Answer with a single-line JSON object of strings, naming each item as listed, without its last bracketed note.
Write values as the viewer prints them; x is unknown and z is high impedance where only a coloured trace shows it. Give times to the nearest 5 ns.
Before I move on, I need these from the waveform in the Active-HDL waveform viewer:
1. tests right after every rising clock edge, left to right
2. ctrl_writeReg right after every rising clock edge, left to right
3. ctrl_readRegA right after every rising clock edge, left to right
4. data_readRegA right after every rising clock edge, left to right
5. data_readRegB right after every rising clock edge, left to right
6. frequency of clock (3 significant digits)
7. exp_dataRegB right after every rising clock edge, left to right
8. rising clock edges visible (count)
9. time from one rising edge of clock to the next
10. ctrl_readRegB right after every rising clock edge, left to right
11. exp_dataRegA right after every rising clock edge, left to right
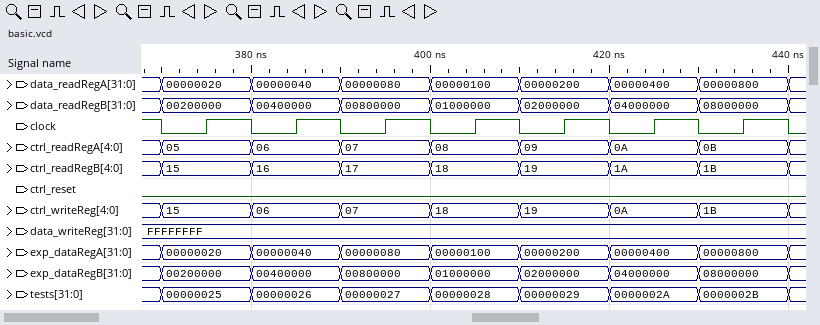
{"tests right after every rising clock edge, left to right": "00000025, 00000026, 00000027, 00000028, 00000029, 0000002A, 0000002B", "ctrl_writeReg right after every rising clock edge, left to right": "15, 06, 07, 18, 19, 0A, 1B", "ctrl_readRegA right after every rising clock edge, left to right": "05, 06, 07, 08, 09, 0A, 0B", "data_readRegA right after every rising clock edge, left to right": "00000020, 00000040, 00000080, 00000100, 00000200, 00000400, 00000800", "data_readRegB right after every rising clock edge, left to right": "00200000, 00400000, 00800000, 01000000, 02000000, 04000000, 08000000", "frequency of clock": "100 MHz", "exp_dataRegB right after every rising clock edge, left to right": "00200000, 00400000, 00800000, 01000000, 02000000, 04000000, 08000000", "rising clock edges visible": "7", "time from one rising edge of clock to the next": "10 ns", "ctrl_readRegB right after every rising clock edge, left to right": "15, 16, 17, 18, 19, 1A, 1B", "exp_dataRegA right after every rising clock edge, left to right": "00000020, 00000040, 00000080, 00000100, 00000200, 00000400, 00000800"}
